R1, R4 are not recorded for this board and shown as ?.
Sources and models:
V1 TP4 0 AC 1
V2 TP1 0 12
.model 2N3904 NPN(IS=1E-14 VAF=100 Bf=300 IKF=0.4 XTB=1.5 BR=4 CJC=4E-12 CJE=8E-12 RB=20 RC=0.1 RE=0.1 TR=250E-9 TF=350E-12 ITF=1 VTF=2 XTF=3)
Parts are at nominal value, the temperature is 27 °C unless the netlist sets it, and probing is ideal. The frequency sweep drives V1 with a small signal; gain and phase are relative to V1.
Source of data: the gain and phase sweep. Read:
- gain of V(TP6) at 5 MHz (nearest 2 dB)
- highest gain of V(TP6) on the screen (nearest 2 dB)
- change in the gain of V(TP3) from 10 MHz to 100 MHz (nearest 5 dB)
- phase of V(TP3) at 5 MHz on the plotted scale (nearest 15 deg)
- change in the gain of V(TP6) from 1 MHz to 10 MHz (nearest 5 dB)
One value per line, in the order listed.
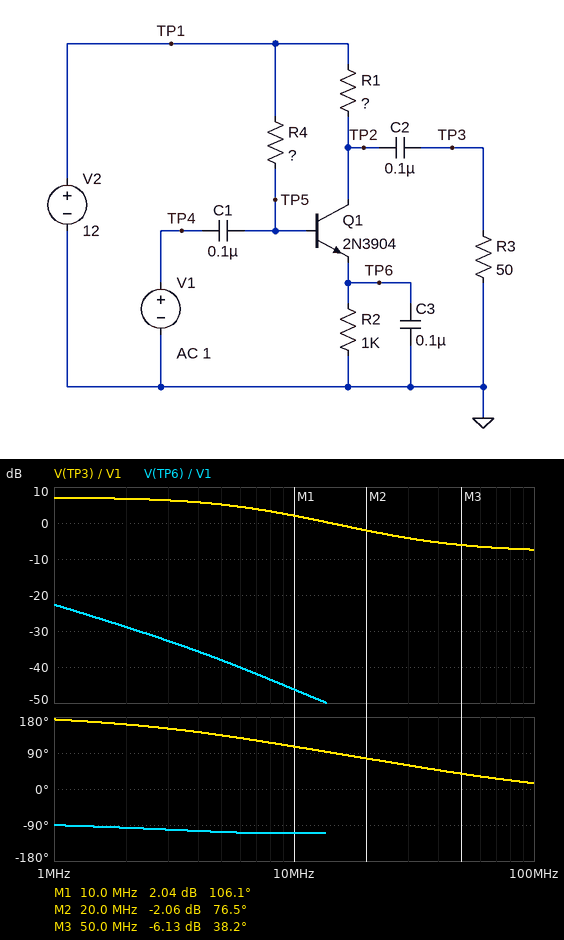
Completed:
-38 dB
-22 dB
-10 dB
135 deg
-25 dB
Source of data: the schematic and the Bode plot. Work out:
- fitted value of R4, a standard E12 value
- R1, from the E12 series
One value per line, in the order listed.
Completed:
1 MΩ
8.2 kΩ
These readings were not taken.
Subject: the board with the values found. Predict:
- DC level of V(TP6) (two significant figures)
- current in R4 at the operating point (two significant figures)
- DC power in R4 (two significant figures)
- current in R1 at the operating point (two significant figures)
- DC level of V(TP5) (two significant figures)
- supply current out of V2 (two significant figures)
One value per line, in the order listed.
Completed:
1.3 V
10 µA
100 µW
1.3 mA
2.0 V
1.3 mA
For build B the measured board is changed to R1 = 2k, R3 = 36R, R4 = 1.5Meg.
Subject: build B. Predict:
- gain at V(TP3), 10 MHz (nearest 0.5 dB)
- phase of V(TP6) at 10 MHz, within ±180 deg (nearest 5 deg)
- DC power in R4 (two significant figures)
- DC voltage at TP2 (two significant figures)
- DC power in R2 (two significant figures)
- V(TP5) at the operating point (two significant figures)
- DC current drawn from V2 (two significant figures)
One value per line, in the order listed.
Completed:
8.5 dB
-90 deg
58 µW
8.1 V
3.9 mW
2.6 V
2.0 mA
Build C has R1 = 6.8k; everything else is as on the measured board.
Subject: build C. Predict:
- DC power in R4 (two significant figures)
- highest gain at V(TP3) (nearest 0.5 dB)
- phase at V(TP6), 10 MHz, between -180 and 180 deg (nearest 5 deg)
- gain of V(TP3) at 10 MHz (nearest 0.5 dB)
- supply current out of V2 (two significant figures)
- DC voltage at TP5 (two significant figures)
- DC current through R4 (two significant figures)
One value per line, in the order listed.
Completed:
96 µW
8.5 dB
-115 deg
4.0 dB
1.5 mA
2.2 V
9.8 µA
